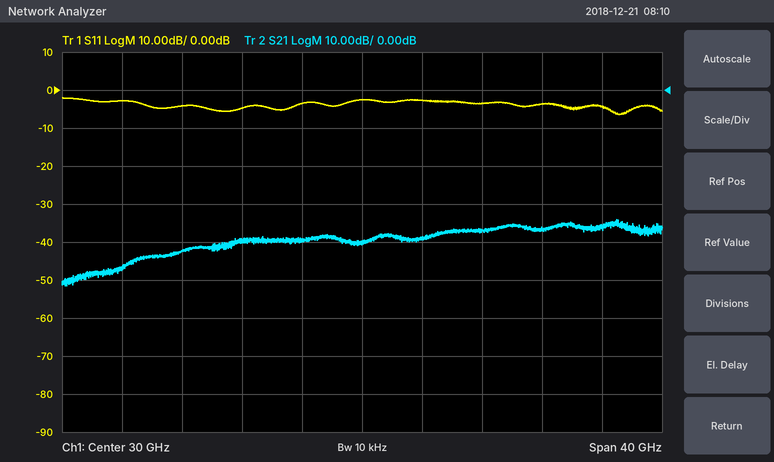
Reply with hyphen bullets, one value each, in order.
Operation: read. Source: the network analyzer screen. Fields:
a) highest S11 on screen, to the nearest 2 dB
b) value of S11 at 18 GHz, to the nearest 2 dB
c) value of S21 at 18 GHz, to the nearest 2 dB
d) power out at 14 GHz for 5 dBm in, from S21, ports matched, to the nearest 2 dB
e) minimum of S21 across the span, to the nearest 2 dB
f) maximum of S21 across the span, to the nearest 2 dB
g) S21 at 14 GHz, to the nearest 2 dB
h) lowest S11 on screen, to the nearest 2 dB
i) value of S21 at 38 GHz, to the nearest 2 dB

- -2 dB
- -4 dB
- -42 dB
- -42 dBm
- -52 dB
- -34 dB
- -46 dB
- -6 dB
- -36 dB
